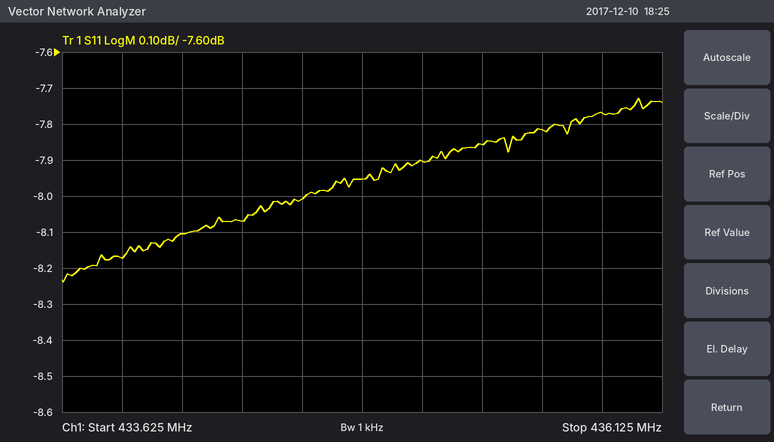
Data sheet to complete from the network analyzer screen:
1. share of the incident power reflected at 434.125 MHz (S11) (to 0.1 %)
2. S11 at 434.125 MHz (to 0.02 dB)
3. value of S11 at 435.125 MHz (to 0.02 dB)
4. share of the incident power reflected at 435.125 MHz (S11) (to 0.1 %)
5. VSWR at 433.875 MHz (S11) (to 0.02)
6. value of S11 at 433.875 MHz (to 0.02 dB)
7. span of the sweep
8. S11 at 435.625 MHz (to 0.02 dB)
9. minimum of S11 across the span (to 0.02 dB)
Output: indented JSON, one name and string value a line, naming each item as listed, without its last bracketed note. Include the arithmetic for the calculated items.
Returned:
{
  "share of the incident power reflected at 434.125 MHz (S11)": "10^(-8.1/10) ≈ 15.5 %",
  "S11 at 434.125 MHz": "-8.10 dB",
  "value of S11 at 435.125 MHz": "-7.90 dB",
  "share of the incident power reflected at 435.125 MHz (S11)": "10^(-7.9/10) ≈ 16.2 %",
  "VSWR at 433.875 MHz (S11)": "|Γ| = 10^(-8.18/20) = 0.3899; VSWR = (1 + 0.3899)/(1 − 0.3899) ≈ 2.28",
  "value of S11 at 433.875 MHz": "-8.18 dB",
  "span of the sweep": "2.5 MHz",
  "S11 at 435.625 MHz": "-7.82 dB",
  "minimum of S11 across the span": "-8.24 dB"
}
